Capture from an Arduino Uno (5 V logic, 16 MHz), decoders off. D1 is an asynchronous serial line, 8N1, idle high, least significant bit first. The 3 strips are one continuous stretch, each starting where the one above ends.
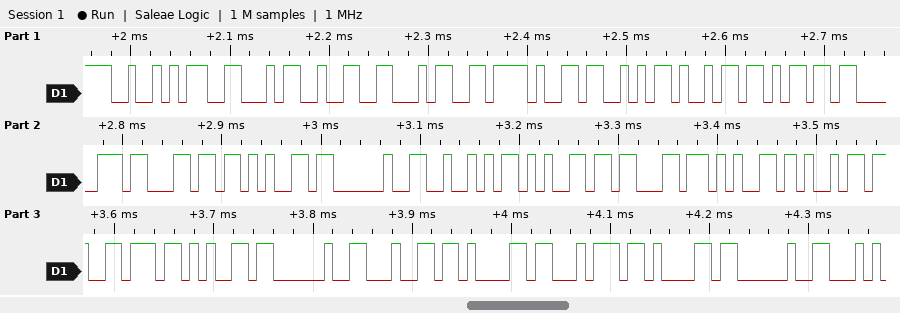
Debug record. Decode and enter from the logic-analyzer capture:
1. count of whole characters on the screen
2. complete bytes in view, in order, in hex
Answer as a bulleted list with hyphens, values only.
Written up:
- 25
- 52 46 32 34 2F 53 69 6D 70 6C 65 20 52 65 63 65 69 76 65 20 64 61 74 61 20
